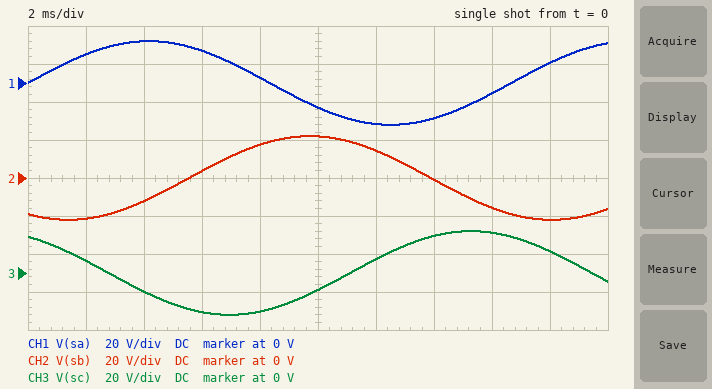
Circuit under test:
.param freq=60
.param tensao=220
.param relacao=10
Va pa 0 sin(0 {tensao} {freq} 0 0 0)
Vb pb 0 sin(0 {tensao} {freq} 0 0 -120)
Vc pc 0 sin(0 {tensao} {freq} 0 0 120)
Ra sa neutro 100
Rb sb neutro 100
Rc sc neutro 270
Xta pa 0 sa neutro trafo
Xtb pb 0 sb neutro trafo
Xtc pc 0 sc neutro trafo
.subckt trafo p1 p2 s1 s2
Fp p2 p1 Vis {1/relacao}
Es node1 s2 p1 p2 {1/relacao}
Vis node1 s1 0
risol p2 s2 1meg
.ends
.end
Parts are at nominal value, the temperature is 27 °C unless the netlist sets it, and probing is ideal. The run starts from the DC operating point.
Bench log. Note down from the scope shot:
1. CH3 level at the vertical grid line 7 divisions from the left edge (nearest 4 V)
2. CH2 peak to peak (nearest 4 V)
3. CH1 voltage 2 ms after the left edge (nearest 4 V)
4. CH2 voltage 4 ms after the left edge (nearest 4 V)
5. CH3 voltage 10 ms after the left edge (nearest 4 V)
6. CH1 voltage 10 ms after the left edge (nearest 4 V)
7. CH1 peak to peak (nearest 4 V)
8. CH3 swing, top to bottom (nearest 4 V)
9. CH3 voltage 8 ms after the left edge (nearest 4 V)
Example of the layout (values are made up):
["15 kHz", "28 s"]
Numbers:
["20 V", "44 V", "16 V", "-12 V", "-8 V", "-12 V", "44 V", "44 V", "-20 V"]
